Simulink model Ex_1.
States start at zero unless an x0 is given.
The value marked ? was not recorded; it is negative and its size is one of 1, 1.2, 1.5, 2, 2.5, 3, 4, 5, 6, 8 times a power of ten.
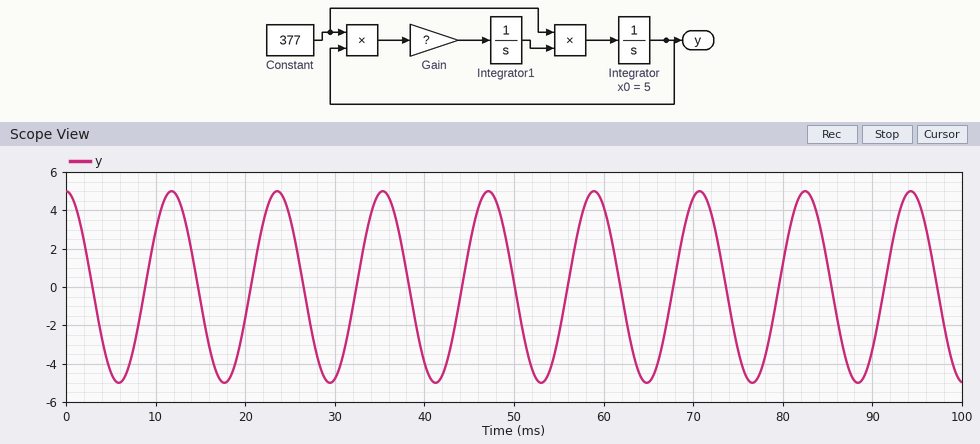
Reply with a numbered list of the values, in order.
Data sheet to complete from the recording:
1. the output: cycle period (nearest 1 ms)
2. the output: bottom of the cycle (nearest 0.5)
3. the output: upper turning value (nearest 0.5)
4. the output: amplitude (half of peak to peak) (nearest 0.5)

1. 12 ms
2. -5.0
3. 5.0
4. 5.0
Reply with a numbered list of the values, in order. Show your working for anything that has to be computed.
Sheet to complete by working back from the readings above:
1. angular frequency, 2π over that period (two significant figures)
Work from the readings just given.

1. 2π / 12 = 0.52 rad/ms
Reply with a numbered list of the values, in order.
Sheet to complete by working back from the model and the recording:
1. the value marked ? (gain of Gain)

1. -2
